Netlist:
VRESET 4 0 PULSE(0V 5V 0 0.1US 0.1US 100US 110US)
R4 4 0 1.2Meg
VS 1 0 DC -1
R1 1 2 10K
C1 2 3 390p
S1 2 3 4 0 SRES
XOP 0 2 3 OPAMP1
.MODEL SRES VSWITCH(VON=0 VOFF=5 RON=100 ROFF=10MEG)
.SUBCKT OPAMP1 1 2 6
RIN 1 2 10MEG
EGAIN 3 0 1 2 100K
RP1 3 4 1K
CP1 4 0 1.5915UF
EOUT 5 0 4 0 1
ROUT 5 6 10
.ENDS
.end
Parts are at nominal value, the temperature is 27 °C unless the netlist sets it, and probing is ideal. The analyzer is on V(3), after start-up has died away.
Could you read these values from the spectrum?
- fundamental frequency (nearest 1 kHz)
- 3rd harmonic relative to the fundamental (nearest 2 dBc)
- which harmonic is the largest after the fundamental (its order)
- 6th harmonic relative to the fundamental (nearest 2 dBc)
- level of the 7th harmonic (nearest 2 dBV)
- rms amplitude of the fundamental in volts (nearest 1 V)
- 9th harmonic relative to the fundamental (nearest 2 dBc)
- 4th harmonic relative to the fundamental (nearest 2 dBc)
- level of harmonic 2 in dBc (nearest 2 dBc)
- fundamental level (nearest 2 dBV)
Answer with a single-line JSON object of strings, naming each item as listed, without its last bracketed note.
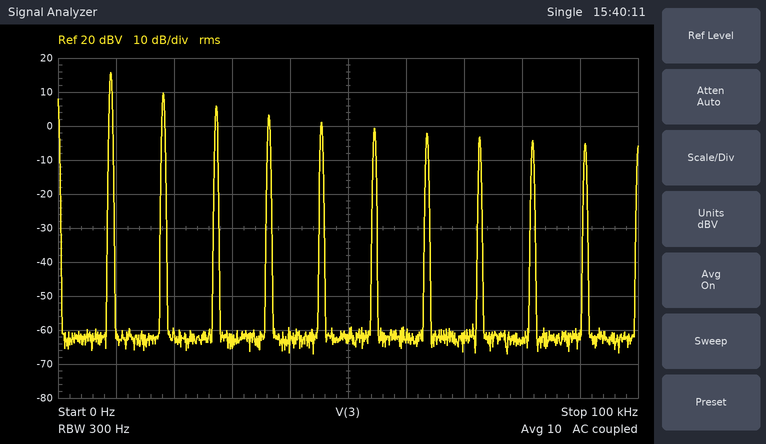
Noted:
{"fundamental frequency": "9 kHz", "3rd harmonic relative to the fundamental": "-10 dBc", "which harmonic is the largest after the fundamental": "2", "6th harmonic relative to the fundamental": "-16 dBc", "level of the 7th harmonic": "-2 dBV", "rms amplitude of the fundamental in volts": "6 V", "9th harmonic relative to the fundamental": "-20 dBc", "4th harmonic relative to the fundamental": "-12 dBc", "level of harmonic 2 in dBc": "-6 dBc", "fundamental level": "16 dBV"}
